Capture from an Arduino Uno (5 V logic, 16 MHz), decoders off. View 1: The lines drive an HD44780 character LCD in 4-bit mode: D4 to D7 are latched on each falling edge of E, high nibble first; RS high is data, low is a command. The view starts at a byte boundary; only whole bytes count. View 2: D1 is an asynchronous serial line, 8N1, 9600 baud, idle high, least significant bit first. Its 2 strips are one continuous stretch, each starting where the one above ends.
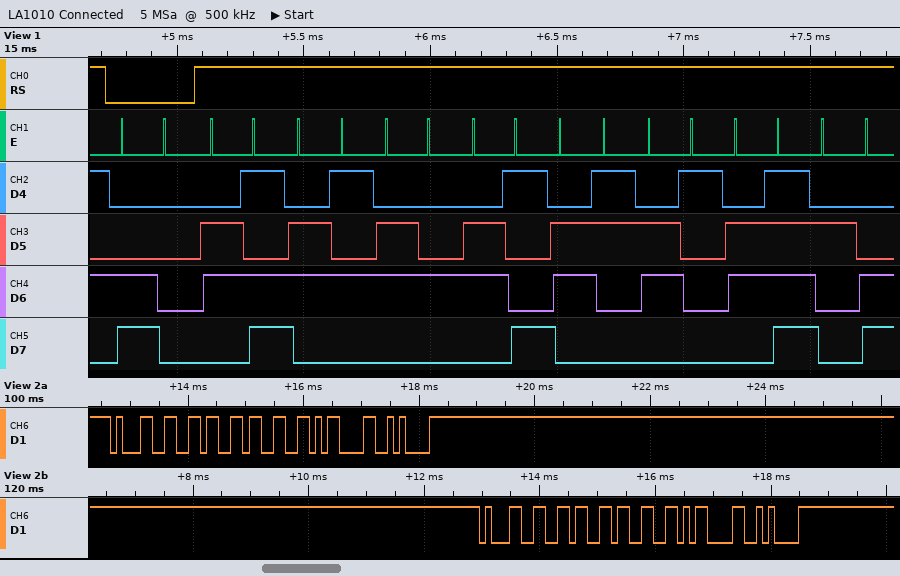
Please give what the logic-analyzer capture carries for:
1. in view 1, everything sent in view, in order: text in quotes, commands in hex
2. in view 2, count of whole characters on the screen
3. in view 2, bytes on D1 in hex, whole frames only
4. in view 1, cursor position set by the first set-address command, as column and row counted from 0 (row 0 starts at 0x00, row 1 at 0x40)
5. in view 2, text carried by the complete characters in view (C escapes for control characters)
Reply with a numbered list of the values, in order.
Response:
1. 0xC0 "medicao,"
2. 10
3. 31 36 33 0D 0A 31 36 33 0D 0A
4. column 0, row 1
5. "163\r\n163\r\n"
